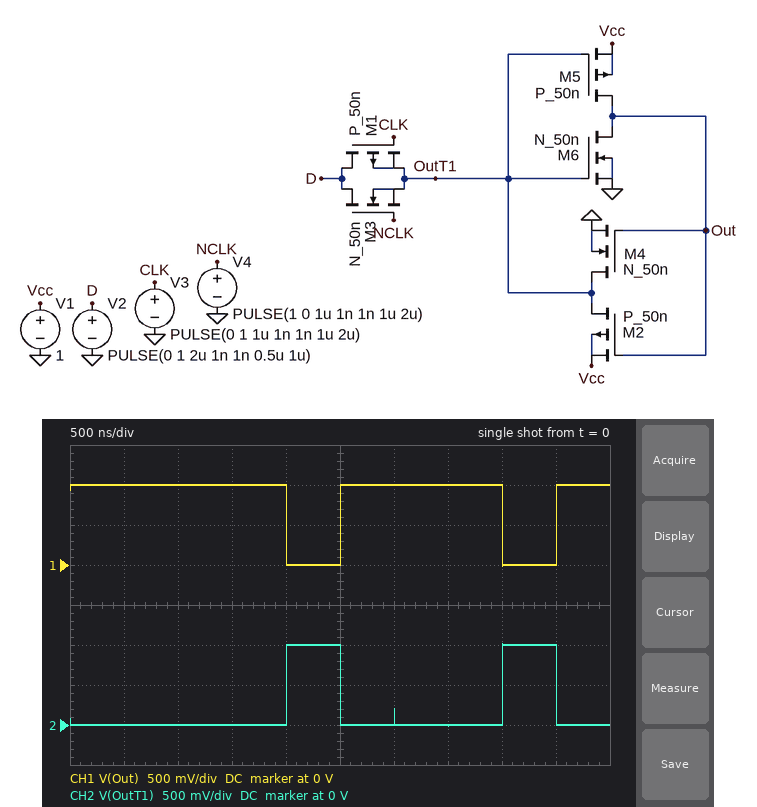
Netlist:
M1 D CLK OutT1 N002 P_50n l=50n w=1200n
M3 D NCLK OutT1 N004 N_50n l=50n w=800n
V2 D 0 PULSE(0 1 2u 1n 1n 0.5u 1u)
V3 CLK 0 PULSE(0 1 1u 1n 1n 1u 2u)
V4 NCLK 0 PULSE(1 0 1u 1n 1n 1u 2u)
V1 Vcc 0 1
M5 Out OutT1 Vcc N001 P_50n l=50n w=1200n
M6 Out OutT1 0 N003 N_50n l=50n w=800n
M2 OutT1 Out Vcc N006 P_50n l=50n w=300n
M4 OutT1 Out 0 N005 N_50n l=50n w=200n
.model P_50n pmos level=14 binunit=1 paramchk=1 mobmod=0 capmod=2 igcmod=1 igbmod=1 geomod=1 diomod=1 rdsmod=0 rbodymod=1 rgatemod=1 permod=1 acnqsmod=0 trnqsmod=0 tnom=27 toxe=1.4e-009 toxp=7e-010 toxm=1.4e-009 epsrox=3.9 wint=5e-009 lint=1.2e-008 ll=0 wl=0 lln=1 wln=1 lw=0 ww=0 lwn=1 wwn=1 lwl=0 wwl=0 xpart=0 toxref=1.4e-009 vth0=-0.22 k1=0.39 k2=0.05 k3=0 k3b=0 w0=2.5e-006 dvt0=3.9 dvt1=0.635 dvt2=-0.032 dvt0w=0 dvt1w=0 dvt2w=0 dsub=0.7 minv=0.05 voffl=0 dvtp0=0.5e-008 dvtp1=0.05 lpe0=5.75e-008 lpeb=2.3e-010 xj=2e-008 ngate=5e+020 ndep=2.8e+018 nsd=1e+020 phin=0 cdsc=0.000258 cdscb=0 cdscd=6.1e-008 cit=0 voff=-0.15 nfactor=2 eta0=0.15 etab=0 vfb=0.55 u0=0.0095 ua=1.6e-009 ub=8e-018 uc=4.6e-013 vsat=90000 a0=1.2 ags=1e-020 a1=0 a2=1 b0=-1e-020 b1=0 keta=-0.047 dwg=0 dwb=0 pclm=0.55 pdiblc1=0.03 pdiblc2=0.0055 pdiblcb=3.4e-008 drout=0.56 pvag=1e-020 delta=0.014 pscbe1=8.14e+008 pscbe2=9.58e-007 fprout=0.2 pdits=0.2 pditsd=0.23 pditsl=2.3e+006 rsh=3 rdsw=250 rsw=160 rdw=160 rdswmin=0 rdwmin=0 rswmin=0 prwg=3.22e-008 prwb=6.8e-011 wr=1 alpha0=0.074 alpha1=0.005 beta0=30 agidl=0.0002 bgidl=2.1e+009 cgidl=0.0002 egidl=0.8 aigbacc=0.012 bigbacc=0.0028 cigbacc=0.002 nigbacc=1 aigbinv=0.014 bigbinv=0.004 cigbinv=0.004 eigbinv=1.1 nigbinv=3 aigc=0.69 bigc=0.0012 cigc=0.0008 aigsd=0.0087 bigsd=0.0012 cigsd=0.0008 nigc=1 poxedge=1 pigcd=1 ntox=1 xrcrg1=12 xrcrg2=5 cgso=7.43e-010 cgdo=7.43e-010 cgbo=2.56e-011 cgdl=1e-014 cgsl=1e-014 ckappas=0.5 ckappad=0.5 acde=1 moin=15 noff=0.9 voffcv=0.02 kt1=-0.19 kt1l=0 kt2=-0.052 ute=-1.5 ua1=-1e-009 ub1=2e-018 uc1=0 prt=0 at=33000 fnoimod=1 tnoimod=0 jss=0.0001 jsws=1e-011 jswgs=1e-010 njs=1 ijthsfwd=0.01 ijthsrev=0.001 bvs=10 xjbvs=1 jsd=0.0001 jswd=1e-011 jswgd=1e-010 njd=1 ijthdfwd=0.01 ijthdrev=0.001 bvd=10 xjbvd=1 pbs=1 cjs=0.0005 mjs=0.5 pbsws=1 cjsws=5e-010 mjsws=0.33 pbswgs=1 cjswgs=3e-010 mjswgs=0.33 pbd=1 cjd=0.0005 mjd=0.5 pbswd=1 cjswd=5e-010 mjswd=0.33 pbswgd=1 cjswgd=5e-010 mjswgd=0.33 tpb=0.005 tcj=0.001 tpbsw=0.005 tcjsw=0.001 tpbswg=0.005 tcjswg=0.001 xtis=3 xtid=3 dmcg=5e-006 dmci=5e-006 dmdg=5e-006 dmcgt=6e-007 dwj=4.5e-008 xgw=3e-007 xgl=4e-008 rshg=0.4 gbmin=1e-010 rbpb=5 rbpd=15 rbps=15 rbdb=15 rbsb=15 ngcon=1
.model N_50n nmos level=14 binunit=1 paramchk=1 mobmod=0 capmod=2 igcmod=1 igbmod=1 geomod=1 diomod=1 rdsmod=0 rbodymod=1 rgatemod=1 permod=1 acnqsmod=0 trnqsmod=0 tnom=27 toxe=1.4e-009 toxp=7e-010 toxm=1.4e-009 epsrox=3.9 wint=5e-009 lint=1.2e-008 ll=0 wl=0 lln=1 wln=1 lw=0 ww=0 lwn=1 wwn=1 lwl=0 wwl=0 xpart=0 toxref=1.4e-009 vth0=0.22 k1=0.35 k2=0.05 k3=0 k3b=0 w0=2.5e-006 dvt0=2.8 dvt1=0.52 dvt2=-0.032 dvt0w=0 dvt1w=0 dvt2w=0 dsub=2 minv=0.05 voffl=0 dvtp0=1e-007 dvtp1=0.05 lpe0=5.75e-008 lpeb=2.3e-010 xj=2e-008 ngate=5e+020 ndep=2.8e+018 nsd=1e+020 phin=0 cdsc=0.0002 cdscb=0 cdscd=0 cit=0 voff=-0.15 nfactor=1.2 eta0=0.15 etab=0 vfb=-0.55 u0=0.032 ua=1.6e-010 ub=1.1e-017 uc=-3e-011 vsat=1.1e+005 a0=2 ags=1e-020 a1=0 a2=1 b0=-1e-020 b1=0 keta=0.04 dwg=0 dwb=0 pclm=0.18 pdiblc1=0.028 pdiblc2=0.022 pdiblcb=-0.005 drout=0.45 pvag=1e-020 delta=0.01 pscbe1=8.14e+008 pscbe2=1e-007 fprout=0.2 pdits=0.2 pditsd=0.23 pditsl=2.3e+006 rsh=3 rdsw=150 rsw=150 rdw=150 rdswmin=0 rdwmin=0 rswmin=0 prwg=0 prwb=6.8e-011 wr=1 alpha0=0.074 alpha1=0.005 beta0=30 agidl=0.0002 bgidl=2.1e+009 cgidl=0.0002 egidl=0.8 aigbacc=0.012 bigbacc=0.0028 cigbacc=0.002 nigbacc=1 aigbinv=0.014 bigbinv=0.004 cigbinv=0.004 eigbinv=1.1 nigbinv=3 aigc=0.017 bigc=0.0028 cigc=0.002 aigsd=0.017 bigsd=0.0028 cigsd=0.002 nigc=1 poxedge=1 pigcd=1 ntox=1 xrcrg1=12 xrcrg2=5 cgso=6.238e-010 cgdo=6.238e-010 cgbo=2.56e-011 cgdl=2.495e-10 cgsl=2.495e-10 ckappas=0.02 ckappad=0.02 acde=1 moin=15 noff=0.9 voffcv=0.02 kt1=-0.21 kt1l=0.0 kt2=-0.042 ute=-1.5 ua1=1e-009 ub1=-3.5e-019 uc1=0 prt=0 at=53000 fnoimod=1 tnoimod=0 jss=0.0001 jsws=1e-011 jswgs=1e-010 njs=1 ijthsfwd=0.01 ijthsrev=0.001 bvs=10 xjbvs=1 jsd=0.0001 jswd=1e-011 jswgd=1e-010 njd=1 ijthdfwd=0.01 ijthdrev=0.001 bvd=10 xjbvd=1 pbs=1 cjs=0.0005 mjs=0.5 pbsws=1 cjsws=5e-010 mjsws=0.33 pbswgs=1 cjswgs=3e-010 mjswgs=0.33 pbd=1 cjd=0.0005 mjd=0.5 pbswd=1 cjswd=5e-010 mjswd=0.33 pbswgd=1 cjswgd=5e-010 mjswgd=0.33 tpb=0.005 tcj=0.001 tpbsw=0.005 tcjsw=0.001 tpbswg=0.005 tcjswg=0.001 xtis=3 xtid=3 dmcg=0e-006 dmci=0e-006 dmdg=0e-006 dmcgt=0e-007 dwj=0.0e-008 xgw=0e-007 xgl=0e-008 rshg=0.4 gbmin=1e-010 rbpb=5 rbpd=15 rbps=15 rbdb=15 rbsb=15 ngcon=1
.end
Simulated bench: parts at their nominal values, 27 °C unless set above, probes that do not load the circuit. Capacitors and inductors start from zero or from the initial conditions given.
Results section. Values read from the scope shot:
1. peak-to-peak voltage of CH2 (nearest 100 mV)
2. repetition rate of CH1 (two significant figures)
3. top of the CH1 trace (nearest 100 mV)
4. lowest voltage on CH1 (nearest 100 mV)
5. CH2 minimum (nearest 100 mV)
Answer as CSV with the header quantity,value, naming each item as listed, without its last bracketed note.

quantity,value
peak-to-peak voltage of CH2,1.0 V
repetition rate of CH1,500 kHz
top of the CH1 trace,1.0 V
lowest voltage on CH1,0 V
CH2 minimum,0 V
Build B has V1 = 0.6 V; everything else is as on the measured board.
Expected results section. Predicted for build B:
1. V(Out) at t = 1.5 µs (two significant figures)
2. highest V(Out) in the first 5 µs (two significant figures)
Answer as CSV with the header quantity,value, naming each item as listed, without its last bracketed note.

quantity,value
V(Out) at t = 1.5 µs,600 mV
highest V(Out) in the first 5 µs,610 mV
